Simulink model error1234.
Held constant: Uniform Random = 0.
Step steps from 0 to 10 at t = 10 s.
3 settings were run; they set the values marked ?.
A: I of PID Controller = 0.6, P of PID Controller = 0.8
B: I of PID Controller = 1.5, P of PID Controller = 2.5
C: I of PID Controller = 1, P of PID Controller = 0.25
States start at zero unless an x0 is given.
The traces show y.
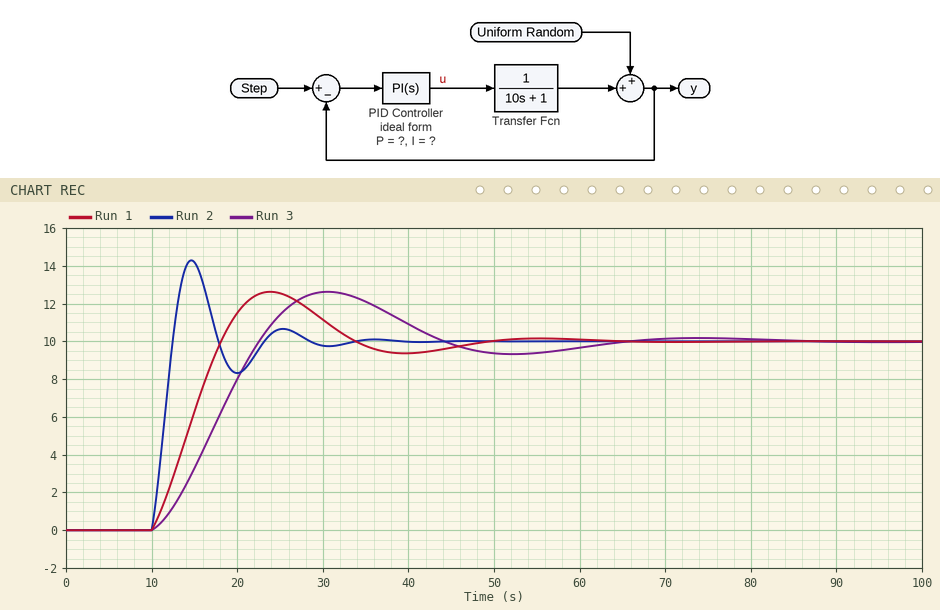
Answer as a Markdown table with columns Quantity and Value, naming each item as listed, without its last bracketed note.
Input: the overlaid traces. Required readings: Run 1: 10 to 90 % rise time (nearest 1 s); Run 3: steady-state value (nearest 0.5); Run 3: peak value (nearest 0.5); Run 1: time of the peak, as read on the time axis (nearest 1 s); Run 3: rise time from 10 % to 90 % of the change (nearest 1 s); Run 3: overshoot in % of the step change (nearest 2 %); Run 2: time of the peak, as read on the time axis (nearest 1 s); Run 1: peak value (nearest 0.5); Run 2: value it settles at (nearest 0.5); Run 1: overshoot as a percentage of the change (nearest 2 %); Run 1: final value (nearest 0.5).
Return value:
| Quantity | Value |
|---|---|
| Run 1: 10 to 90 % rise time | 6 s |
| Run 3: steady-state value | 10.0 |
| Run 3: peak value | 12.5 |
| Run 1: time of the peak, as read on the time axis | 24 s |
| Run 3: rise time from 10 % to 90 % of the change | 9 s |
| Run 3: overshoot in % of the step change | 26 % |
| Run 2: time of the peak, as read on the time axis | 15 s |
| Run 1: peak value | 12.5 |
| Run 2: value it settles at | 10.0 |
| Run 1: overshoot as a percentage of the change | 26 % |
| Run 1: final value | 10.0 |
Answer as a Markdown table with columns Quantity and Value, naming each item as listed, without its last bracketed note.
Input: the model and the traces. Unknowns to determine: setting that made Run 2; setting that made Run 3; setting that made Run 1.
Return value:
| Quantity | Value |
|---|---|
| setting that made Run 2 | B |
| setting that made Run 3 | C |
| setting that made Run 1 | A |
